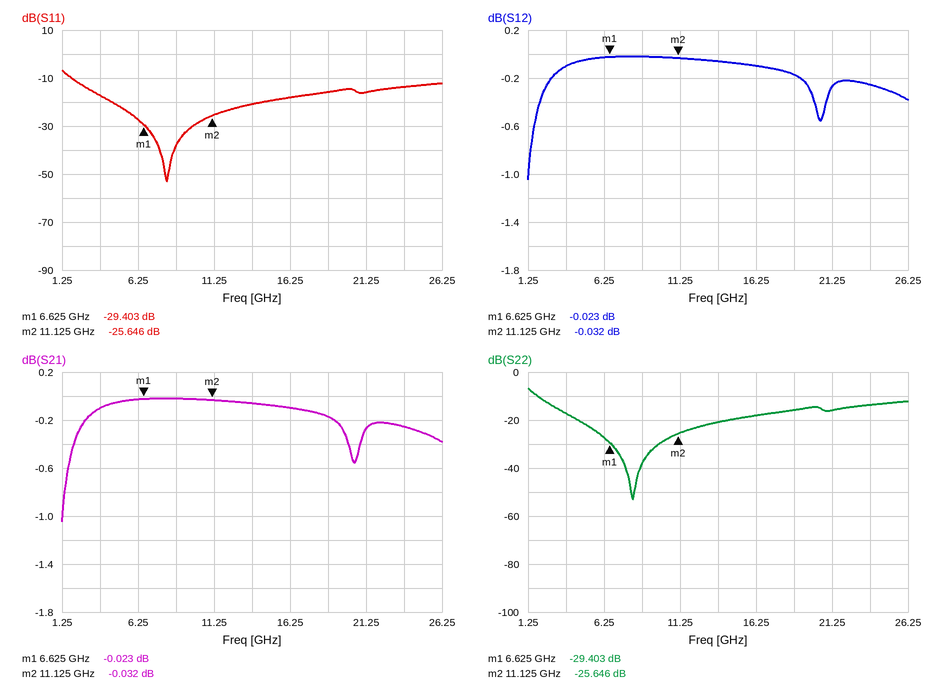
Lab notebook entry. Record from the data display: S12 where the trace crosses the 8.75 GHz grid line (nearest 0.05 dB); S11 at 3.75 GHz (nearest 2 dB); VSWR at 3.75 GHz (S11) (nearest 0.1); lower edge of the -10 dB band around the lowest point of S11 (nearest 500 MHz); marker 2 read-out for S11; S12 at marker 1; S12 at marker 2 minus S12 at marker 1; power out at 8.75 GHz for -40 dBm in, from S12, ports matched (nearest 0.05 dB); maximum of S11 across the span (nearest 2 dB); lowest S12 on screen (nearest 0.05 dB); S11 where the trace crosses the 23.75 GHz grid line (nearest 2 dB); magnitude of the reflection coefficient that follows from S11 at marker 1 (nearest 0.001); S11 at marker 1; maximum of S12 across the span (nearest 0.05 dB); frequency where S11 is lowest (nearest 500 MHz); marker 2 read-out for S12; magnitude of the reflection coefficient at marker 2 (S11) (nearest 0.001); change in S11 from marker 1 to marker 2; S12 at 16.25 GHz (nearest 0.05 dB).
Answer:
0.00 dB
-18 dB
1.3
2.0 GHz
-25.646 dB
-0.023 dB
-0.009 dB
-40.00 dBm
-6 dB
-1.05 dB
-14 dB
0.034
-29.403 dB
0.00 dB
8.0 GHz
-0.032 dB
0.052
3.757 dB
-0.10 dB
